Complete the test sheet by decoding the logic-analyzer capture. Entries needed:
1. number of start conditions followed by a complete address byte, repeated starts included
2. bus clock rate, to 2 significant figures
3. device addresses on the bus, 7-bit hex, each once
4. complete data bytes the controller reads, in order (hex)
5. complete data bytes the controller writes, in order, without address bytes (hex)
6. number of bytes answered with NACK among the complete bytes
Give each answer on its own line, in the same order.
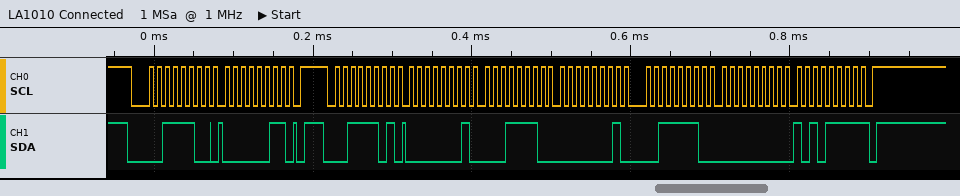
2
100 kHz
0x1E
01 1E 01 3E 00 AF
03
1
